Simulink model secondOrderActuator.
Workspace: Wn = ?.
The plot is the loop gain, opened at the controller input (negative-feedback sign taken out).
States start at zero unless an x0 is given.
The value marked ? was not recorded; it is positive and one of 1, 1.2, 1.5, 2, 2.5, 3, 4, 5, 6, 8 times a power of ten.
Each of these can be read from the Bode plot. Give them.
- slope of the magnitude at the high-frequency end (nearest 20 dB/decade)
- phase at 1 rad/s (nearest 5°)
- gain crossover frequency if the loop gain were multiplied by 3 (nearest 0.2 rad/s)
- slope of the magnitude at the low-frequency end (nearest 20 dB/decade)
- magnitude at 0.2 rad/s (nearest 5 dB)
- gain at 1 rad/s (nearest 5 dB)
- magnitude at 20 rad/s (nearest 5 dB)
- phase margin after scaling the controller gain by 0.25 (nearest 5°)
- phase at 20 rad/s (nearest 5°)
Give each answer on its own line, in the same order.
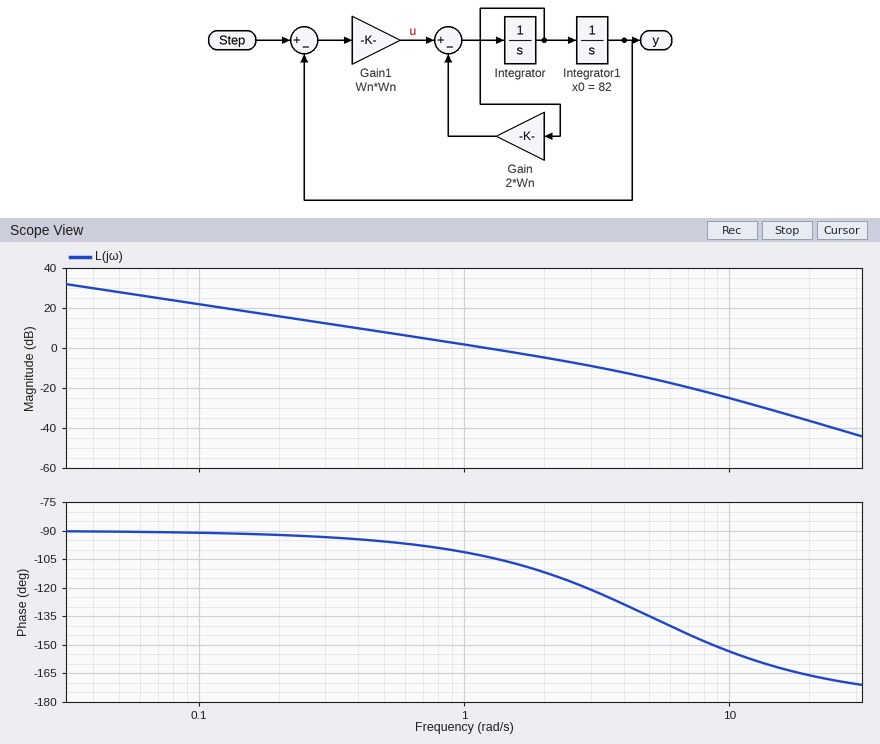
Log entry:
-40 dB/decade
-100°
3.2 rad/s
-20 dB/decade
15 dB
0 dB
-35 dB
85°
-165°
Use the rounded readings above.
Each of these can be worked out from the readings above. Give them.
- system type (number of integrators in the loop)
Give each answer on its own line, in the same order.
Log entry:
1
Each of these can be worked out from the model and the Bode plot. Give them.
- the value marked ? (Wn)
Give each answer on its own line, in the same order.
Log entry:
2.5
